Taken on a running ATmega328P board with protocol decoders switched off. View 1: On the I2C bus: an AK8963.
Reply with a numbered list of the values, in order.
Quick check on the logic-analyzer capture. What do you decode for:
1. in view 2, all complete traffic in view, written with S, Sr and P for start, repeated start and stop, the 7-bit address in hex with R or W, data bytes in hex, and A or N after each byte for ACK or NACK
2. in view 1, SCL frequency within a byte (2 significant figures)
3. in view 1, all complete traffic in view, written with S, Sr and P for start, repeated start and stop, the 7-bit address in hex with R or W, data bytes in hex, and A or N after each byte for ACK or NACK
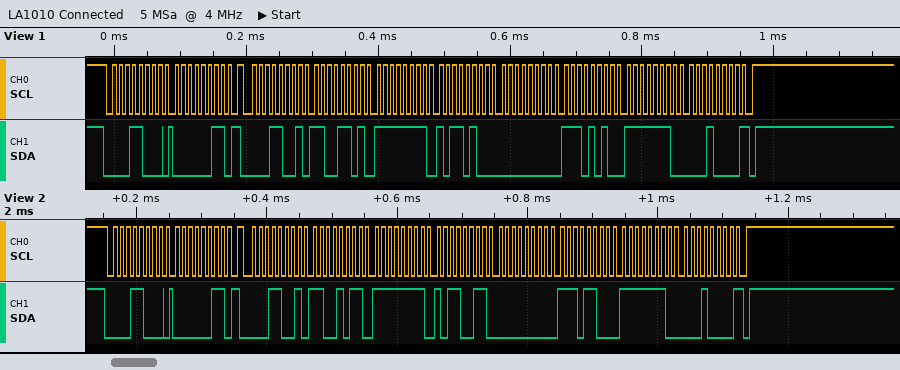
1. S 0CW A 03 A Sr 0CR A CB A FF A B3 A 00 A EC A FE A 10 N P
2. 100 kHz
3. S 0CW A 03 A Sr 0CR A CD A FF A B4 A 00 A EA A FE A 10 N P
